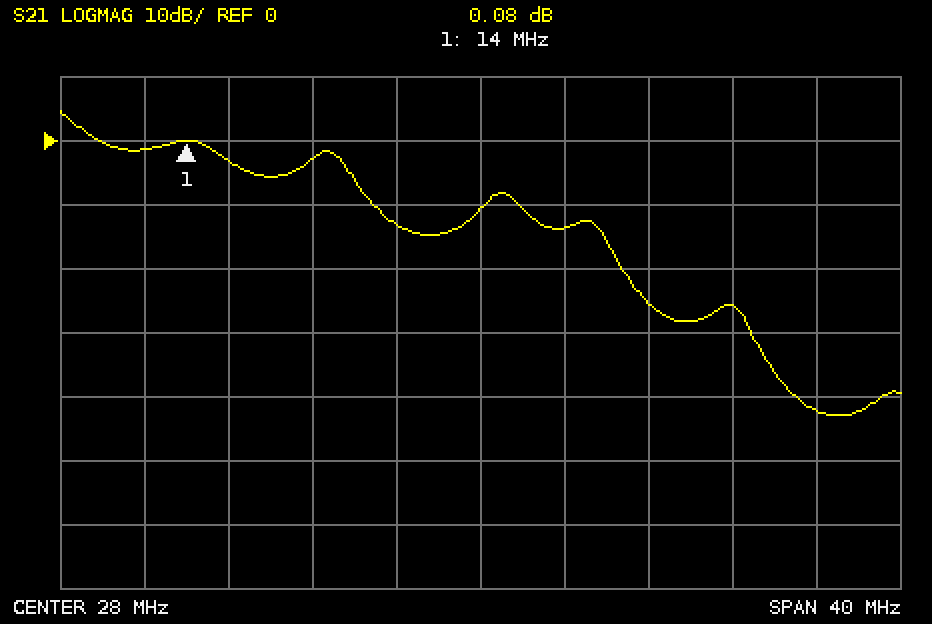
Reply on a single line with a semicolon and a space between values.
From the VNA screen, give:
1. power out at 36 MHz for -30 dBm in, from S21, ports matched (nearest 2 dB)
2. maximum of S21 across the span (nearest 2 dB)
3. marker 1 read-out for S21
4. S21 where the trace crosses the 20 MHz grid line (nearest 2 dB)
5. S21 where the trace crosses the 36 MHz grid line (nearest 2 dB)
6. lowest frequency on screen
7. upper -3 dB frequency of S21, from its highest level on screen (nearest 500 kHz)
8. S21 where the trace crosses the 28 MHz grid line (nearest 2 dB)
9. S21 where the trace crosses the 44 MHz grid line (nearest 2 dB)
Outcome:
-56 dBm; 4 dB; 0.08 dB; -2 dB; -26 dB; 8 MHz; 9.0 MHz; -10 dB; -42 dB
